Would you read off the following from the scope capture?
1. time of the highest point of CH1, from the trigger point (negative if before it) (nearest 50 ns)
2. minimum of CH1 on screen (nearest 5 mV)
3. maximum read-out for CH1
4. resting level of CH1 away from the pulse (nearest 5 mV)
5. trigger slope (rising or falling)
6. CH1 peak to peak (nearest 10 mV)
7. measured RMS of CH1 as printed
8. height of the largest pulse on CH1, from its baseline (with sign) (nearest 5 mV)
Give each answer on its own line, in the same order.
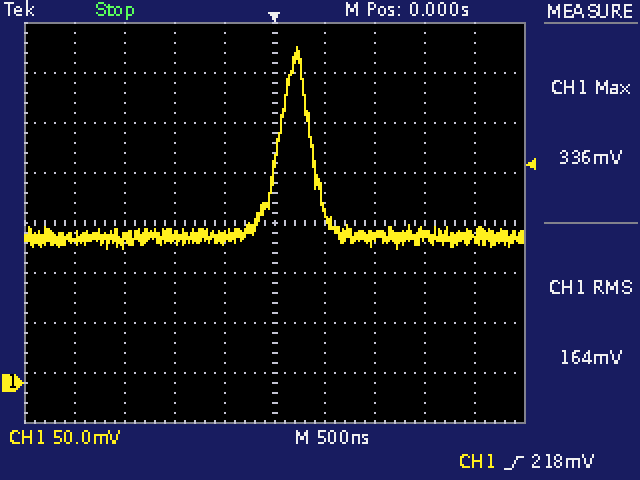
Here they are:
+250 ns
135 mV
336 mV
145 mV
rising
200 mV
164 mV
+190 mV
